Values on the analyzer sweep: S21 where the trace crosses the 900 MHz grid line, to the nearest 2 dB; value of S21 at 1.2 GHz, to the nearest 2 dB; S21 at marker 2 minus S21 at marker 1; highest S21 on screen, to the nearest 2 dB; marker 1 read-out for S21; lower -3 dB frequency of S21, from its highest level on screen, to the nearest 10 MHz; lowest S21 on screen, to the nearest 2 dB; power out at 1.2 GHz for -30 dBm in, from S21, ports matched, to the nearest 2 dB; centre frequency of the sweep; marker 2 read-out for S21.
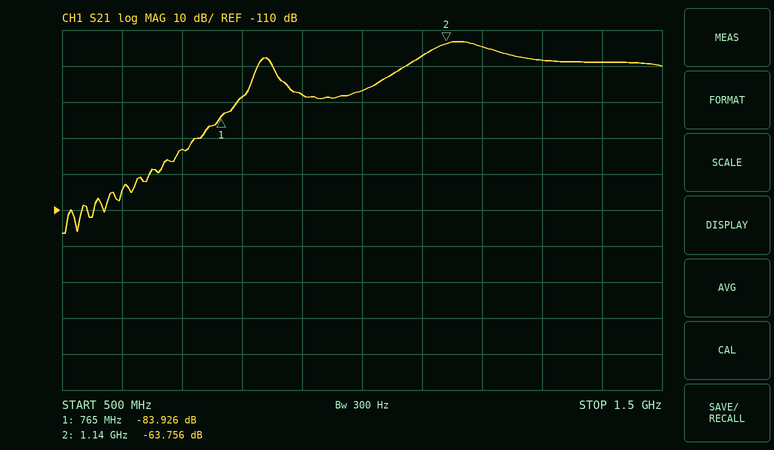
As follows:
-78 dB
-64 dB
20.170 dB
-64 dB
-83.926 dB
1.11 GHz
-116 dB
-94 dBm
1 GHz
-63.756 dB
